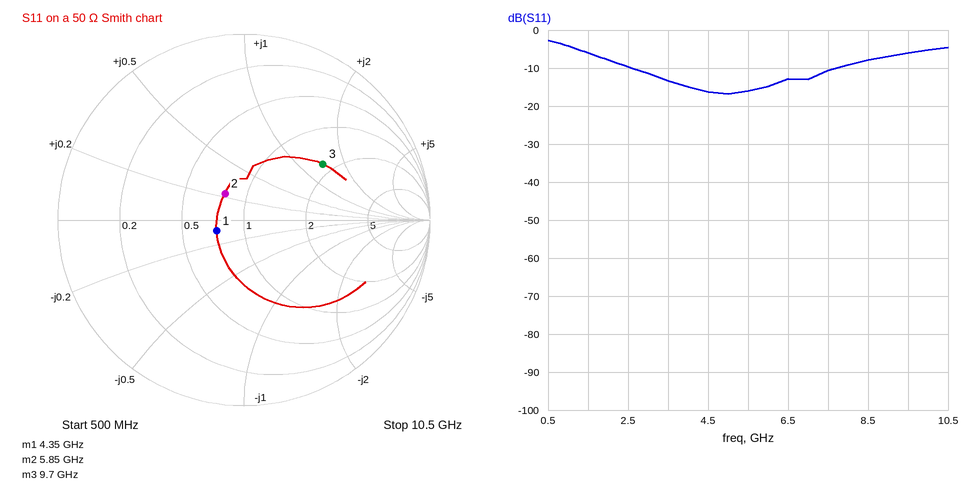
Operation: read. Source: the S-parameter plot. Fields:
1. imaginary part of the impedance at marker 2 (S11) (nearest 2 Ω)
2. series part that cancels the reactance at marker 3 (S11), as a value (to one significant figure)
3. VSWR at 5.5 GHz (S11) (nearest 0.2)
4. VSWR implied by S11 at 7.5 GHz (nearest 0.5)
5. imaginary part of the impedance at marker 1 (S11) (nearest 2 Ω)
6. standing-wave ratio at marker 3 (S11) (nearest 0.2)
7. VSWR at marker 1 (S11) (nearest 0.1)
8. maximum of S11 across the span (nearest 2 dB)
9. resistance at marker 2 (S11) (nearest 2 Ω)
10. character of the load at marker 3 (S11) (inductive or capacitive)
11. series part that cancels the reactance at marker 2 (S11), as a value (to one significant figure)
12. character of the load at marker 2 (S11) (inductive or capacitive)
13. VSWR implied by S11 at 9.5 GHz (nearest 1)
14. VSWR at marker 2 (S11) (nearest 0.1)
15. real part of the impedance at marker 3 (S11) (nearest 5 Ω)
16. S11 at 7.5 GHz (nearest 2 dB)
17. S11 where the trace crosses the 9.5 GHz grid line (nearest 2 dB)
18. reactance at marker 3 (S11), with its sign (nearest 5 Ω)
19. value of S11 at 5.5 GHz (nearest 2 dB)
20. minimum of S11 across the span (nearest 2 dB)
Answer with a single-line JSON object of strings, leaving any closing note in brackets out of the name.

{"imaginary part of the impedance at marker 2 (S11)": "+12 Ω", "series part that cancels the reactance at marker 3 (S11), as a value": "200 fF", "VSWR at 5.5 GHz (S11)": "1.4", "VSWR implied by S11 at 7.5 GHz": "2.0", "imaginary part of the impedance at marker 1 (S11)": "-4 Ω", "standing-wave ratio at marker 3 (S11)": "3.2", "VSWR at marker 1 (S11)": "1.4", "maximum of S11 across the span": "-2 dB", "resistance at marker 2 (S11)": "40 Ω", "character of the load at marker 3 (S11)": "inductive", "series part that cancels the reactance at marker 2 (S11), as a value": "2 pF", "character of the load at marker 2 (S11)": "inductive", "VSWR implied by S11 at 9.5 GHz": "3", "VSWR at marker 2 (S11)": "1.4", "real part of the impedance at marker 3 (S11)": "85 Ω", "S11 at 7.5 GHz": "-10 dB", "S11 where the trace crosses the 9.5 GHz grid line": "-6 dB", "reactance at marker 3 (S11), with its sign": "+70 Ω", "value of S11 at 5.5 GHz": "-16 dB", "minimum of S11 across the span": "-16 dB"}
